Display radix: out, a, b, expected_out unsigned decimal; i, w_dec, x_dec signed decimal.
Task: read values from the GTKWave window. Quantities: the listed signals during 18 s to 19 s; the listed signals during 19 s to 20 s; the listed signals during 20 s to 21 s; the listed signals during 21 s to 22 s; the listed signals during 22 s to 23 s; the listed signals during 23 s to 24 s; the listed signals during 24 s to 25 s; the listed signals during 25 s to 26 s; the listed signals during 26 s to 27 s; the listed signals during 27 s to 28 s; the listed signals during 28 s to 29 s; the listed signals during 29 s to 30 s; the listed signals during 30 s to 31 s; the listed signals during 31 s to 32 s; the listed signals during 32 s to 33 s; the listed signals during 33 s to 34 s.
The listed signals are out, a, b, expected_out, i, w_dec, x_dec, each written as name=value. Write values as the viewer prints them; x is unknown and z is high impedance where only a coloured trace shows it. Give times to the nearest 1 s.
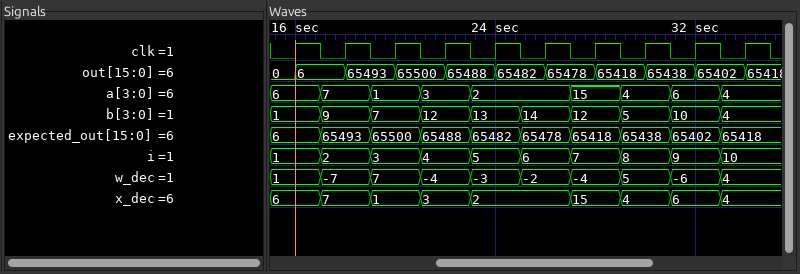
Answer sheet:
out=65493, a=7, b=9, expected_out=65493, i=2, w_dec=-7, x_dec=7
out=65493, a=1, b=7, expected_out=65500, i=3, w_dec=7, x_dec=1
out=65500, a=1, b=7, expected_out=65500, i=3, w_dec=7, x_dec=1
out=65500, a=3, b=12, expected_out=65488, i=4, w_dec=-4, x_dec=3
out=65488, a=3, b=12, expected_out=65488, i=4, w_dec=-4, x_dec=3
out=65488, a=2, b=13, expected_out=65482, i=5, w_dec=-3, x_dec=2
out=65482, a=2, b=13, expected_out=65482, i=5, w_dec=-3, x_dec=2
out=65482, a=2, b=14, expected_out=65478, i=6, w_dec=-2, x_dec=2
out=65478, a=2, b=14, expected_out=65478, i=6, w_dec=-2, x_dec=2
out=65478, a=15, b=12, expected_out=65418, i=7, w_dec=-4, x_dec=15
out=65418, a=15, b=12, expected_out=65418, i=7, w_dec=-4, x_dec=15
out=65418, a=4, b=5, expected_out=65438, i=8, w_dec=5, x_dec=4
out=65438, a=4, b=5, expected_out=65438, i=8, w_dec=5, x_dec=4
out=65438, a=6, b=10, expected_out=65402, i=9, w_dec=-6, x_dec=6
out=65402, a=6, b=10, expected_out=65402, i=9, w_dec=-6, x_dec=6
out=65402, a=4, b=4, expected_out=65418, i=10, w_dec=4, x_dec=4
